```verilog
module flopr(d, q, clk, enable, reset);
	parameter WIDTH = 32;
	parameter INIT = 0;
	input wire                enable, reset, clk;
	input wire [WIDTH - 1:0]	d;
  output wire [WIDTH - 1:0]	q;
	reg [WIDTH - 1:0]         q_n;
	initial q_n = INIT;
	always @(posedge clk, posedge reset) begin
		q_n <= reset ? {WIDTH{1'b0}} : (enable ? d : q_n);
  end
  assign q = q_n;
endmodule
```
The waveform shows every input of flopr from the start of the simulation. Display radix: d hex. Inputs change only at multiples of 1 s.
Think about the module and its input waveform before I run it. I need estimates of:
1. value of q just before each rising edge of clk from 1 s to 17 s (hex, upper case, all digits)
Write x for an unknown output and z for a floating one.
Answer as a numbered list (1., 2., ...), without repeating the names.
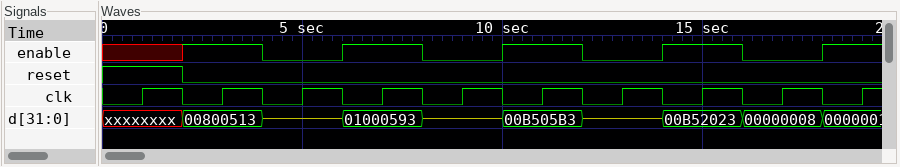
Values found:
1. 00000000, 00000000, 00800513, 00800513, 01000593, 01000593, 00B505B3, 00B505B3, 00B52023
